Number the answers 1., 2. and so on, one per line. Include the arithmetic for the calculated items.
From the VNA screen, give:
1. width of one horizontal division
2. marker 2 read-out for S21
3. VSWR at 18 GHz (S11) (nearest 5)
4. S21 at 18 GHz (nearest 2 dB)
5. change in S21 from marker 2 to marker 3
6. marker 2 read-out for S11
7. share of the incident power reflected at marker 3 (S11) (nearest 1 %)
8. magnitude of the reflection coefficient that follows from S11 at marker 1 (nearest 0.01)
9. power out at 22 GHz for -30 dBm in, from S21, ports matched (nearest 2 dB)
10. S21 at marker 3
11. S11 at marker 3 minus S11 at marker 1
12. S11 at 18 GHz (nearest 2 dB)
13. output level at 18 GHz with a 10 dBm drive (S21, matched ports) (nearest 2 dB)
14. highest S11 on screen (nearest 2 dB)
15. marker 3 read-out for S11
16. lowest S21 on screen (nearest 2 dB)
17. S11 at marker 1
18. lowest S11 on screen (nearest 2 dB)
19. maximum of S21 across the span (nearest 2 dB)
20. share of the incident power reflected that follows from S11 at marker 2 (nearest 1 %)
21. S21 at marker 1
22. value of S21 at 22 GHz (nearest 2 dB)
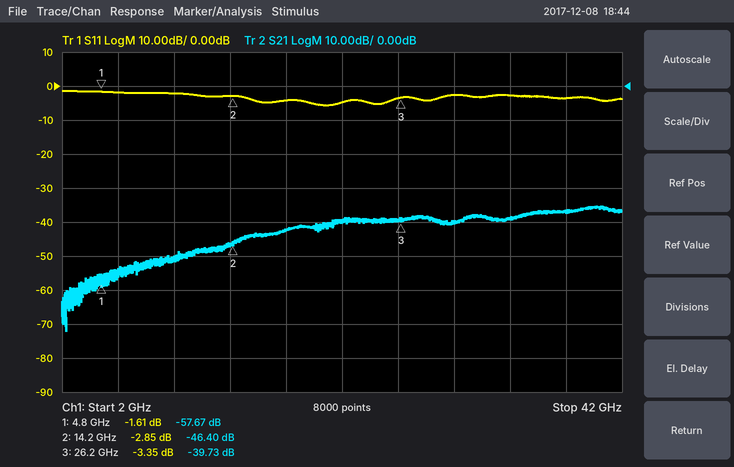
1. 4 GHz
2. -46.40 dB
3. |Γ| = 10^(-4/20) = 0.6310; VSWR = (1 + 0.6310)/(1 − 0.6310) ≈ 4.42, so 5 to the nearest 5
4. -42 dB
5. -39.73 − (-46.4) = 6.67 dB
6. -2.85 dB
7. 10^(-3.35/10) ≈ 46 %
8. 10^(-1.61/20) ≈ 0.83
9. -30 dBm + (-40 dB) = -70 dBm
10. -39.73 dB
11. -3.35 − (-1.61) = -1.74 dB
12. -4 dB
13. 10 dBm + (-42 dB) = -32 dBm
14. -2 dB
15. -3.35 dB
16. -72 dB
17. -1.61 dB
18. -6 dB
19. -36 dB
20. 10^(-2.85/10) ≈ 52 %
21. -57.67 dB
22. -40 dB
